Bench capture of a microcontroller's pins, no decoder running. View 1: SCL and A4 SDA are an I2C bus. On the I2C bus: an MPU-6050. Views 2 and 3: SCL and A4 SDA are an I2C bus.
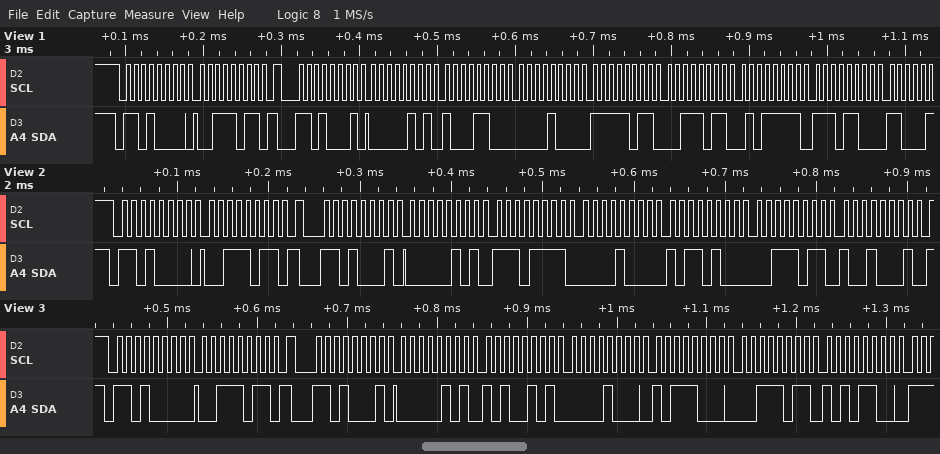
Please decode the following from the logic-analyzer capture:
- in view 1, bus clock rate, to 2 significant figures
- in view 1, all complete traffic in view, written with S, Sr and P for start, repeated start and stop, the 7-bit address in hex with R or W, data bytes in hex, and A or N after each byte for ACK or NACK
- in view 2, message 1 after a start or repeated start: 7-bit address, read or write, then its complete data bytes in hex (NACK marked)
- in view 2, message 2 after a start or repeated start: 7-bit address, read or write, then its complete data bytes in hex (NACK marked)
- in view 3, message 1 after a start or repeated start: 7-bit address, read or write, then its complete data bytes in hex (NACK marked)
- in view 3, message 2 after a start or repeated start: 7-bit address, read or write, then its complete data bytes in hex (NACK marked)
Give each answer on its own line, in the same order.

100 kHz
S 68W A 3B A Sr 68R A 05 A 8C A 08 A FB A 3B A 5F A EC A
0x68 write: 3B
0x68 read: 05 EF 08 B4 3B 91
0x68 write: 3B
0x68 read: 05 A5 08 B8 3B AC
